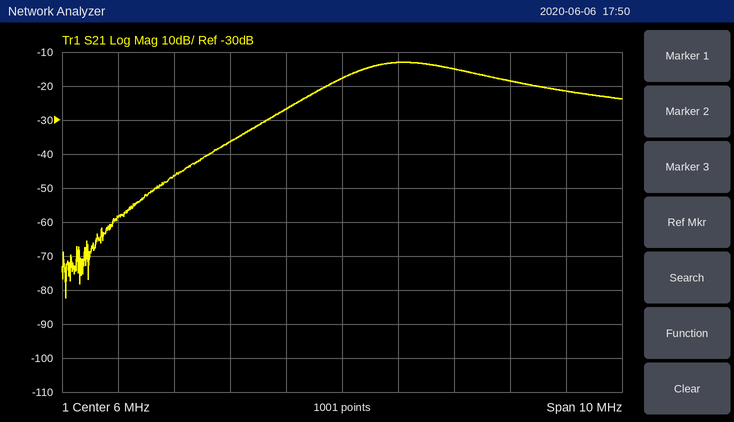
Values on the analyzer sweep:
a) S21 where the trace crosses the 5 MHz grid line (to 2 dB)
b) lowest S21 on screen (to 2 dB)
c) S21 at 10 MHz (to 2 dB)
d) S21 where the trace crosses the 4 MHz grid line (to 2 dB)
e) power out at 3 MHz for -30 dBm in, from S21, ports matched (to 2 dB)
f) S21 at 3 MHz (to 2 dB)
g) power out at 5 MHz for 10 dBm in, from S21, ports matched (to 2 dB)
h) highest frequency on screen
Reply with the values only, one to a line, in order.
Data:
-26 dB
-82 dB
-22 dB
-36 dB
-76 dBm
-46 dB
-16 dBm
11 MHz
